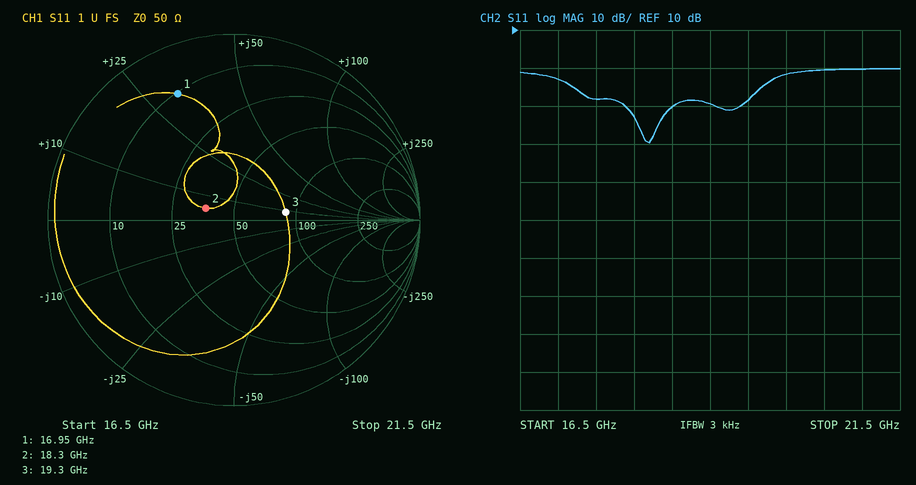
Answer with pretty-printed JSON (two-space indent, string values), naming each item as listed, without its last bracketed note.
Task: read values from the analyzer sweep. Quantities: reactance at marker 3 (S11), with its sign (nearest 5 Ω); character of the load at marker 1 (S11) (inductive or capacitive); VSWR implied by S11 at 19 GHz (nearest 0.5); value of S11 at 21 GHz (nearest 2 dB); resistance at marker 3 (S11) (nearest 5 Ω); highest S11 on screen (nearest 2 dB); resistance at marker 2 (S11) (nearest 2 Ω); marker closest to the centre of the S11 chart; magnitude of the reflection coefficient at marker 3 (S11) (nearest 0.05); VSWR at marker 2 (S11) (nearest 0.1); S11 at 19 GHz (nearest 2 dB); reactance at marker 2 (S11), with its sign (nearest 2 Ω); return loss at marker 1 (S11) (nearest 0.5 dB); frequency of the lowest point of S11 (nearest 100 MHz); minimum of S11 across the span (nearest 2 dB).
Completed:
{
  "reactance at marker 3 (S11), with its sign": "+10 Ω",
  "character of the load at marker 1 (S11)": "inductive",
  "VSWR implied by S11 at 19 GHz": "2.0",
  "value of S11 at 21 GHz": "0 dB",
  "resistance at marker 3 (S11)": "90 Ω",
  "highest S11 on screen": "0 dB",
  "resistance at marker 2 (S11)": "36 Ω",
  "marker closest to the centre of the S11 chart": "marker 2",
  "magnitude of the reflection coefficient at marker 3 (S11)": "0.30",
  "VSWR at marker 2 (S11)": "1.4",
  "S11 at 19 GHz": "-10 dB",
  "reactance at marker 2 (S11), with its sign": "+4 Ω",
  "return loss at marker 1 (S11)": "2.5 dB",
  "frequency of the lowest point of S11": "18.2 GHz",
  "minimum of S11 across the span": "-20 dB"
}
